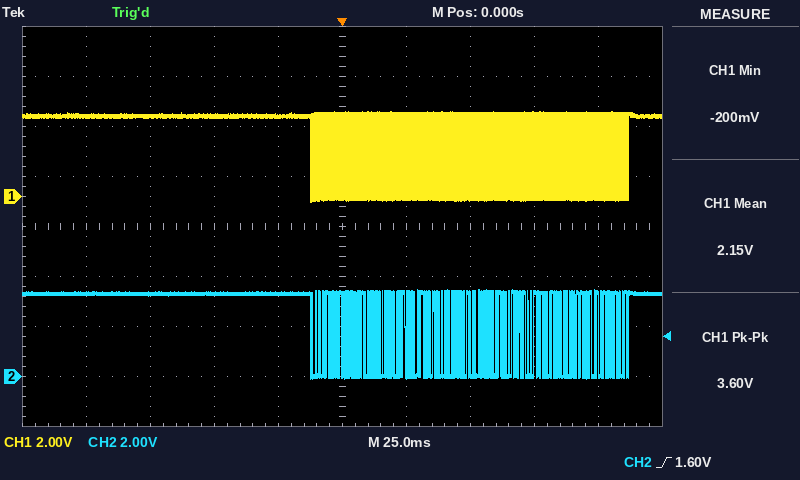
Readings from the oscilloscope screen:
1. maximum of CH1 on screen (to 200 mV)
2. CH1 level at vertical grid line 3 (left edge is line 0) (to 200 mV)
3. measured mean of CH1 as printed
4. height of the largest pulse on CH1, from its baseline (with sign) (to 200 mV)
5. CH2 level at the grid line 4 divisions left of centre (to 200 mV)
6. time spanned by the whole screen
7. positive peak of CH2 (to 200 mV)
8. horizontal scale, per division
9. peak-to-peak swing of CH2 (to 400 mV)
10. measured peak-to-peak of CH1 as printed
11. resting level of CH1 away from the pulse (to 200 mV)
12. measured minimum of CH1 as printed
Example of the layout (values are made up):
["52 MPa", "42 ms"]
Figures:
["3.4 V", "3.2 V", "2.15 V", "-3.4 V", "3.4 V", "250 ms", "3.4 V", "25 ms", "3.6 V", "3.60 V", "3.2 V", "-200 mV"]
